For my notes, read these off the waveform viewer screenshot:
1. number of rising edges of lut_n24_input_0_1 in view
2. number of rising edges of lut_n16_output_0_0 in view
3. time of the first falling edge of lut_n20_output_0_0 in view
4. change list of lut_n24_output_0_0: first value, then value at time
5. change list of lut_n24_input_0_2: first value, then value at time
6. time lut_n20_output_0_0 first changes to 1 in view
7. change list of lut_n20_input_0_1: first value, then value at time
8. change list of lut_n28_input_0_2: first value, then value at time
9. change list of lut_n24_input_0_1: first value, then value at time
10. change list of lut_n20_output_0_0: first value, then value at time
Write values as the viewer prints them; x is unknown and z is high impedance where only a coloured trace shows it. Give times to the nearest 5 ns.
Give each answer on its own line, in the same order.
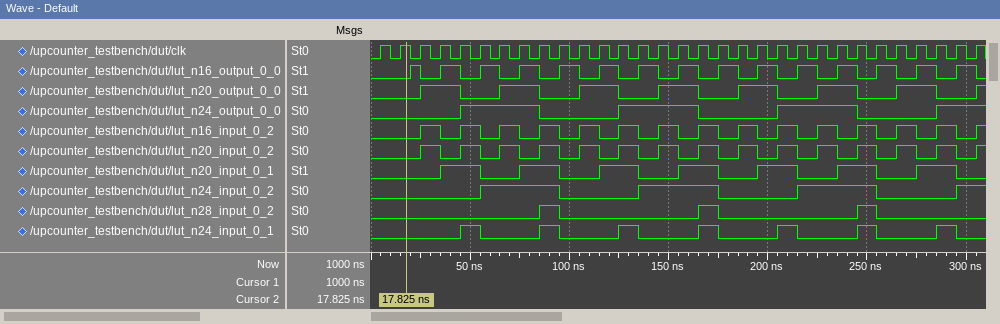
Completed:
7
15
45 ns
0, 1 at 45 ns, 0 at 85 ns, 1 at 125 ns, 0 at 165 ns, 1 at 205 ns, 0 at 245 ns, 1 at 285 ns
0, 1 at 55 ns, 0 at 95 ns, 1 at 135 ns, 0 at 175 ns, 1 at 215 ns, 0 at 255 ns, 1 at 295 ns
25 ns
0, 1 at 35 ns, 0 at 55 ns, 1 at 75 ns, 0 at 95 ns, 1 at 115 ns, 0 at 135 ns, 1 at 155 ns, 0 at 175 ns, 1 at 195 ns, 0 at 215 ns, 1 at 235 ns, 0 at 255 ns, 1 at 275 ns, 0 at 295 ns
0, 1 at 85 ns, 0 at 95 ns, 1 at 165 ns, 0 at 175 ns, 1 at 245 ns, 0 at 255 ns
0, 1 at 45 ns, 0 at 55 ns, 1 at 85 ns, 0 at 95 ns, 1 at 125 ns, 0 at 135 ns, 1 at 165 ns, 0 at 175 ns, 1 at 205 ns, 0 at 215 ns, 1 at 245 ns, 0 at 255 ns, 1 at 285 ns, 0 at 295 ns
0, 1 at 25 ns, 0 at 45 ns, 1 at 65 ns, 0 at 85 ns, 1 at 105 ns, 0 at 125 ns, 1 at 145 ns, 0 at 165 ns, 1 at 185 ns, 0 at 205 ns, 1 at 225 ns, 0 at 245 ns, 1 at 265 ns, 0 at 285 ns, 1 at 305 ns
